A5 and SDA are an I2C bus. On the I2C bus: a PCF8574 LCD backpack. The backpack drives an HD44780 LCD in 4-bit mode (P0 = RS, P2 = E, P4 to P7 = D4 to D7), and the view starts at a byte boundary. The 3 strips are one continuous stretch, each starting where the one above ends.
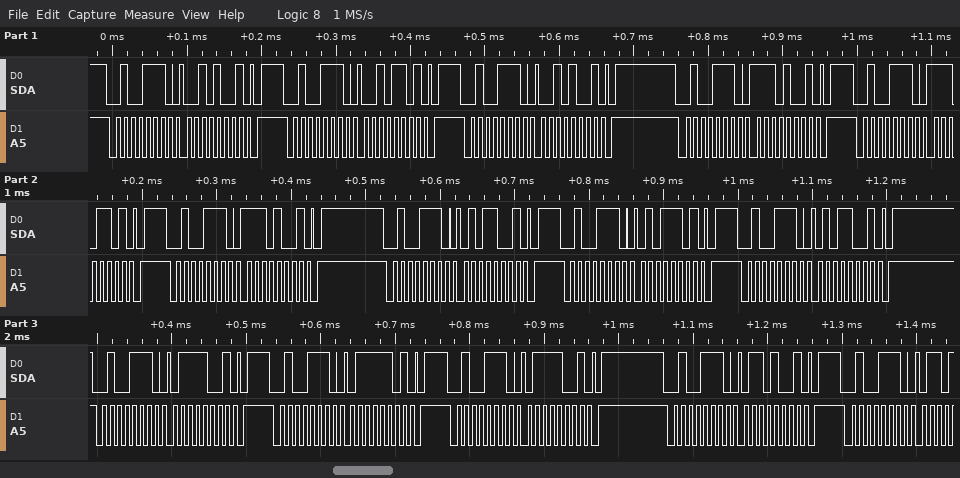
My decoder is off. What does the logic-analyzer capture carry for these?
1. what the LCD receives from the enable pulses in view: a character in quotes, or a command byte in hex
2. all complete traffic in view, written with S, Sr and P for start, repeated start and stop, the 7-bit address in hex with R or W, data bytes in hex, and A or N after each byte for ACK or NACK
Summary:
'.' 'W'
S 27W A 29 A P S 27W A 2D A P S 27W A 29 A P S 27W A E9 A P S 27W A ED A P S 27W A E9 A P S 27W A 59 A P S 27W A 5D A P S 27W A 59 A P S 27W A 79 A P S 27W A 7D A P S 27W A 79 A P S 27W A 69 A P S 27W A
